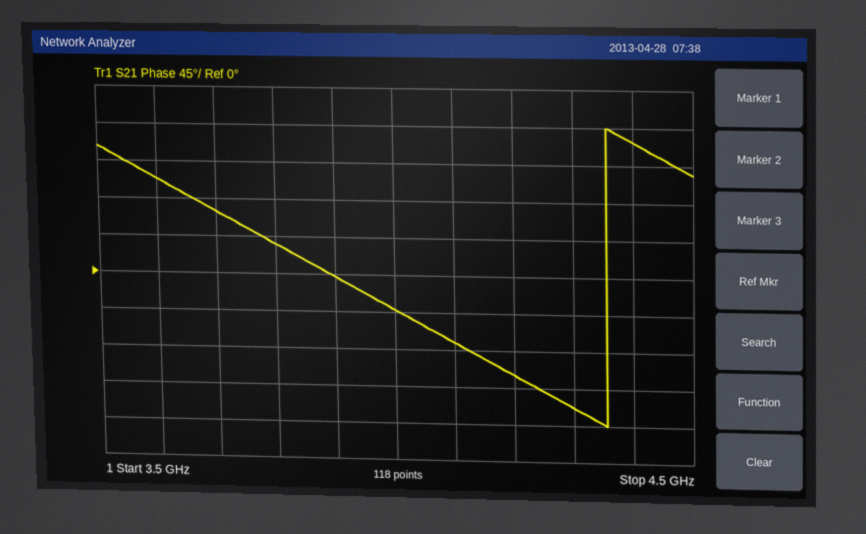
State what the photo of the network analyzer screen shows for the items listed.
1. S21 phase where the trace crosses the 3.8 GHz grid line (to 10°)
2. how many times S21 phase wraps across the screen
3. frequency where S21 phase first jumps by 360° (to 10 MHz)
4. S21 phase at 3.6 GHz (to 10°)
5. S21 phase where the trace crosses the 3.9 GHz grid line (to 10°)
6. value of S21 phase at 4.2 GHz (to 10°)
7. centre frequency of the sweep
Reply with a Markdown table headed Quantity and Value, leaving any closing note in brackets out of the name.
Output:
| Quantity | Value |
|---|---|
| S21 phase where the trace crosses the 3.8 GHz grid line | 40° |
| how many times S21 phase wraps across the screen | 1 |
| frequency where S21 phase first jumps by 360° | 4.36 GHz |
| S21 phase at 3.6 GHz | 110° |
| S21 phase where the trace crosses the 3.9 GHz grid line | 0° |
| value of S21 phase at 4.2 GHz | -120° |
| centre frequency of the sweep | 4 GHz |
